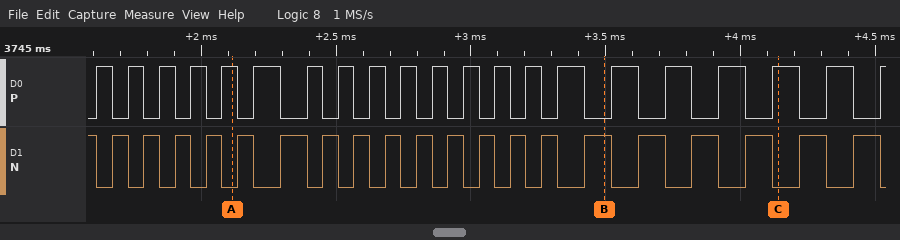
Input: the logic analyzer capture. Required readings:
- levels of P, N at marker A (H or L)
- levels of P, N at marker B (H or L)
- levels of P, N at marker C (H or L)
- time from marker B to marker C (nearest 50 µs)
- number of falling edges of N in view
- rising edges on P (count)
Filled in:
P=H, N=L
P=L, N=H
P=H, N=L
650 µs
21
21
